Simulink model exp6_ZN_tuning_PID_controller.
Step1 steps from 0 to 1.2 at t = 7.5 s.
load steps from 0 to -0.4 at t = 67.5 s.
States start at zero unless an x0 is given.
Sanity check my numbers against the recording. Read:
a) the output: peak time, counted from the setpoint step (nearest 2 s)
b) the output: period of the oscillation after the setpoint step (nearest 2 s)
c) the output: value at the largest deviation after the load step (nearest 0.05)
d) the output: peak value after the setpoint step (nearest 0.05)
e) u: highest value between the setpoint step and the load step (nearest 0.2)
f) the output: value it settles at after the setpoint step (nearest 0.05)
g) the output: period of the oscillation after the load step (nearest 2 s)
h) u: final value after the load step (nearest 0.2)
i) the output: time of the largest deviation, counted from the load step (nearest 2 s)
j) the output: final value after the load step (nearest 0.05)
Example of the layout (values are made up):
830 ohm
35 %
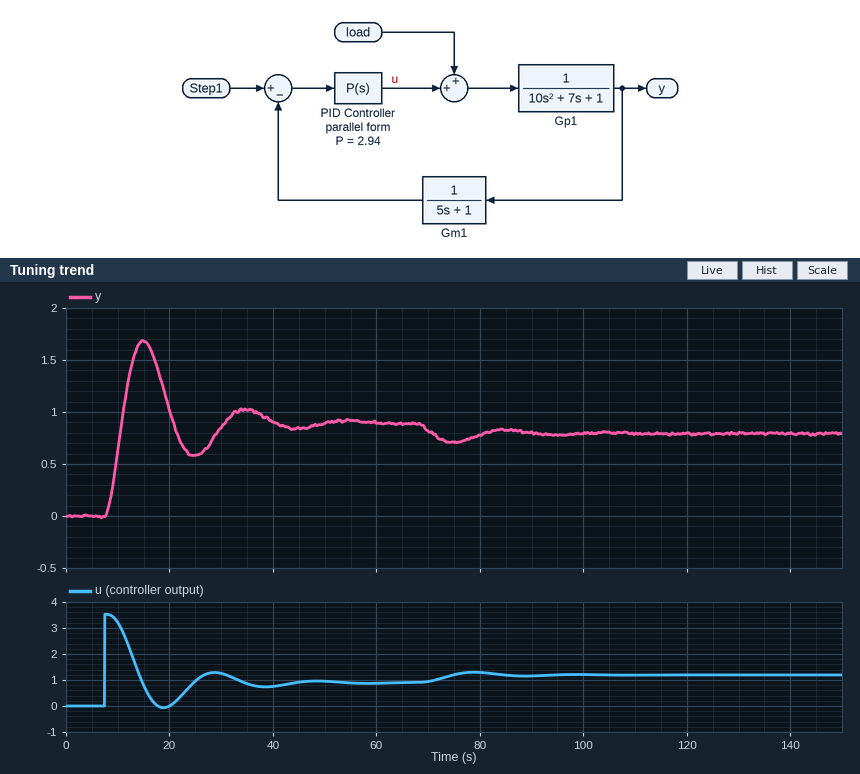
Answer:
8 s
20 s
0.70
1.70
3.6
0.90
20 s
1.2
8 s
0.80
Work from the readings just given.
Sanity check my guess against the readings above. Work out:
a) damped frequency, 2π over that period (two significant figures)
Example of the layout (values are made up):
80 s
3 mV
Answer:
0.31 rad/s
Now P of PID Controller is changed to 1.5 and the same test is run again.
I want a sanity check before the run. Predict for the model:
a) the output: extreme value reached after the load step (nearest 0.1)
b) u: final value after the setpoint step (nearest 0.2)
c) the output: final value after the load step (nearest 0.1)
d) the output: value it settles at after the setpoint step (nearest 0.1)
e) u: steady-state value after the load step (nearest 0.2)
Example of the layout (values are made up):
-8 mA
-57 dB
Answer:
0.5
0.8
0.6
0.7
1.0
